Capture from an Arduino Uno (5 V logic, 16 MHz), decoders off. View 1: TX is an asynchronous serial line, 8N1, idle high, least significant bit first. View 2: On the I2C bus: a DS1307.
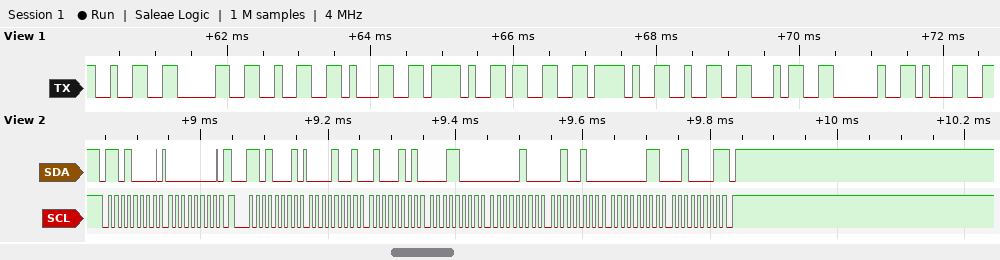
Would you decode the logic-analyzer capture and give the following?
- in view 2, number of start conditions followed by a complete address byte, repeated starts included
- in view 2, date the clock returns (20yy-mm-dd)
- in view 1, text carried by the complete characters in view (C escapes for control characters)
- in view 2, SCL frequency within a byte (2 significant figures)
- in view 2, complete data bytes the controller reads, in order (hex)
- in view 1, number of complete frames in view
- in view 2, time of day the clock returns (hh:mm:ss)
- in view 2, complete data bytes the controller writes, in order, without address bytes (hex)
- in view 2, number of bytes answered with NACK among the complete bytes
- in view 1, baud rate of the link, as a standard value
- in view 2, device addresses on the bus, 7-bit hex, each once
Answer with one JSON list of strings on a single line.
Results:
["2", "2021-03-24", "\"2021/3/24 1\"", "100 kHz", "09 45 18 04 24 03 21", "11", "18:45:09", "00", "1", "9600 baud", "0x68"]
